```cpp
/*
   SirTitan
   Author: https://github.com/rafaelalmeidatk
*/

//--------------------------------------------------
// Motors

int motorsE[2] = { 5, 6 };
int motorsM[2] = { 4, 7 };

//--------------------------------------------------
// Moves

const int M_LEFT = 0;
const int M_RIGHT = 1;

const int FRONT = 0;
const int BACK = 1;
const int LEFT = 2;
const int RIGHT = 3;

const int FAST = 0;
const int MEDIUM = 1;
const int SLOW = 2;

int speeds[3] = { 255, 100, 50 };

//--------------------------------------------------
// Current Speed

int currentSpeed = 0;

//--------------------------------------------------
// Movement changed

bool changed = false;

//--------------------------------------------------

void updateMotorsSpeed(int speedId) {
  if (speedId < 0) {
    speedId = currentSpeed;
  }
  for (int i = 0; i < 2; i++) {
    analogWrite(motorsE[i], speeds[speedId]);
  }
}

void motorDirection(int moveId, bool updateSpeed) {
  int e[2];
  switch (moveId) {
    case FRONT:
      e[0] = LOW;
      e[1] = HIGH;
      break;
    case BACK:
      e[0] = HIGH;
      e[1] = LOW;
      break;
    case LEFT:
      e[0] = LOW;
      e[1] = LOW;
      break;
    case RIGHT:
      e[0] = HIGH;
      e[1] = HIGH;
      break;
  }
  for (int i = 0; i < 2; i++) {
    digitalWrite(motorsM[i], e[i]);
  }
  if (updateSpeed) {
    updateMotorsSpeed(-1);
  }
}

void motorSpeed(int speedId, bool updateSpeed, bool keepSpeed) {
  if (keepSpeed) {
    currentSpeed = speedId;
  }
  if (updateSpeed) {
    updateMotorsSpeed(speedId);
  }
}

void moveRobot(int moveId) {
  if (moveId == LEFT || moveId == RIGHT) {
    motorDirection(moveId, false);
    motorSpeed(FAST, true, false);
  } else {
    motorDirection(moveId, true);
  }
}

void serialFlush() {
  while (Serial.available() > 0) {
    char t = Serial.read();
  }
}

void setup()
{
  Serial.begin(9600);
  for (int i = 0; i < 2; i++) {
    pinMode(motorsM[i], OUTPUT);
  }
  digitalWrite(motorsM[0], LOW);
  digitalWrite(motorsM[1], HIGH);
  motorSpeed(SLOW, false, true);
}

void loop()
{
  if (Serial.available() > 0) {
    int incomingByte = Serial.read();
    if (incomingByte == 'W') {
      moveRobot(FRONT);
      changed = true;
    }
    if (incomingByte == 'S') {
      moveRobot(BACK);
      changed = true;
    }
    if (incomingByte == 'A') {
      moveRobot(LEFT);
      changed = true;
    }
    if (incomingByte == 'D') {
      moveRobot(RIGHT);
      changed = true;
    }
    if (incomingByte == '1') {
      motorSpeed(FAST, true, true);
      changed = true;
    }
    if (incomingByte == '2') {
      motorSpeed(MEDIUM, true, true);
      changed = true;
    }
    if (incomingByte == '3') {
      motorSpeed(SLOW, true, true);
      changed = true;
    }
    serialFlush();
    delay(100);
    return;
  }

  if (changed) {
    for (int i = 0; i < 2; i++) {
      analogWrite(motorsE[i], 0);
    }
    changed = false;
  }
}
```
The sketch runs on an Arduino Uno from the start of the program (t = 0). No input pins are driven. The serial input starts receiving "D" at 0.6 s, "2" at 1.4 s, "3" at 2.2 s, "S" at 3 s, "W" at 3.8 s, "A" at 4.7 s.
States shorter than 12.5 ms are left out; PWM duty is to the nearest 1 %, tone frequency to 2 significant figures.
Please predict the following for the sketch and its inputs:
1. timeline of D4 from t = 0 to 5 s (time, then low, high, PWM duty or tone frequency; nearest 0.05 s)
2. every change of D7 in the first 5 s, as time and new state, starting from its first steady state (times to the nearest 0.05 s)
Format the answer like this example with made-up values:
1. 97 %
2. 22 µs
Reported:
1. 0 s low; 0.6 s high; 3.8 s low
2. 0 s high; 3 s low; 3.8 s high; 4.7 s low
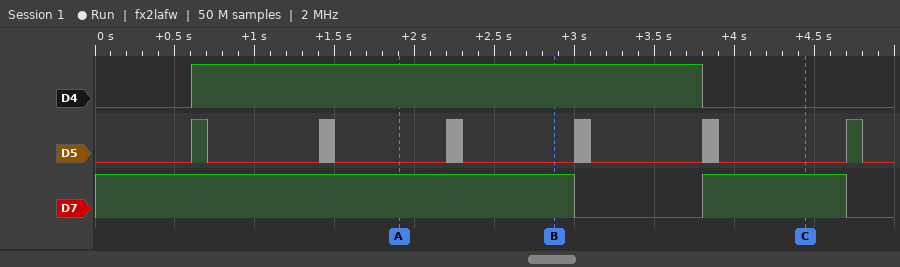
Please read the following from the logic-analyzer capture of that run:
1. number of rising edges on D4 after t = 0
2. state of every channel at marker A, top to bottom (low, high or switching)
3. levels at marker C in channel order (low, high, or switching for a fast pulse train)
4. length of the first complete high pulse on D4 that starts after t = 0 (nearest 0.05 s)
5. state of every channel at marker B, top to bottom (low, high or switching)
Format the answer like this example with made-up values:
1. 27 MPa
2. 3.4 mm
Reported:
1. 1
2. D4 high, D5 low, D7 high
3. D4 low, D5 low, D7 high
4. 3.20 s
5. D4 high, D5 low, D7 high
